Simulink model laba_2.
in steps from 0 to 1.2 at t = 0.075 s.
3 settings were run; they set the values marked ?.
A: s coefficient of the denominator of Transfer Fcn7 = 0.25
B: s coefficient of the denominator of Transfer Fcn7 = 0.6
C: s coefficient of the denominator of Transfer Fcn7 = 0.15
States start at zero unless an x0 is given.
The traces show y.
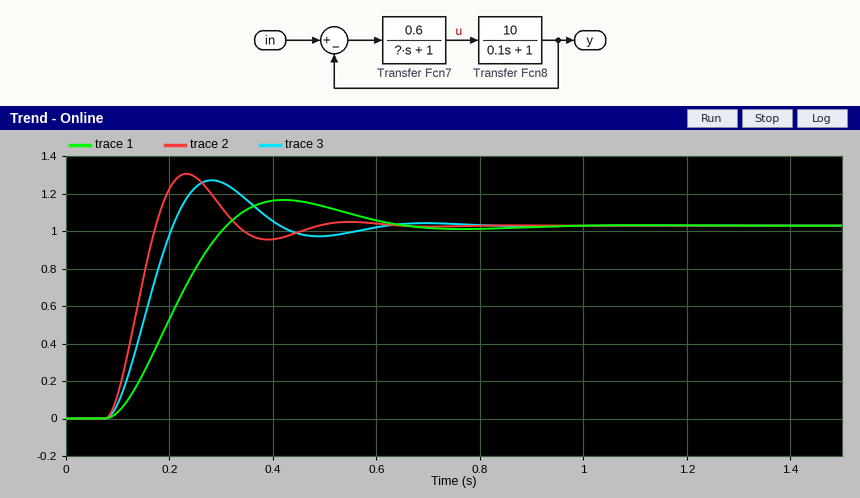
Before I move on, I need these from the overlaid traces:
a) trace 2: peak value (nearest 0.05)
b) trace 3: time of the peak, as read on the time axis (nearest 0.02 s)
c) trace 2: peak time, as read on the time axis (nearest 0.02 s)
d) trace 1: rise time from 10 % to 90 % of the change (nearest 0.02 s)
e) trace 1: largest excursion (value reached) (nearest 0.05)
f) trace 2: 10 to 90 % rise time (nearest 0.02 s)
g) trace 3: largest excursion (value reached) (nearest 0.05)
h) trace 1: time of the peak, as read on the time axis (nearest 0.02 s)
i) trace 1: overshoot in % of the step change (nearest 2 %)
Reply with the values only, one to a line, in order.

1.30
0.28 s
0.24 s
0.16 s
1.15
0.06 s
1.25
0.42 s
14 %
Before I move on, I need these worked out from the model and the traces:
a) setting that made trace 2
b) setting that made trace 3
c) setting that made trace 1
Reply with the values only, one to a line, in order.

C
A
B
